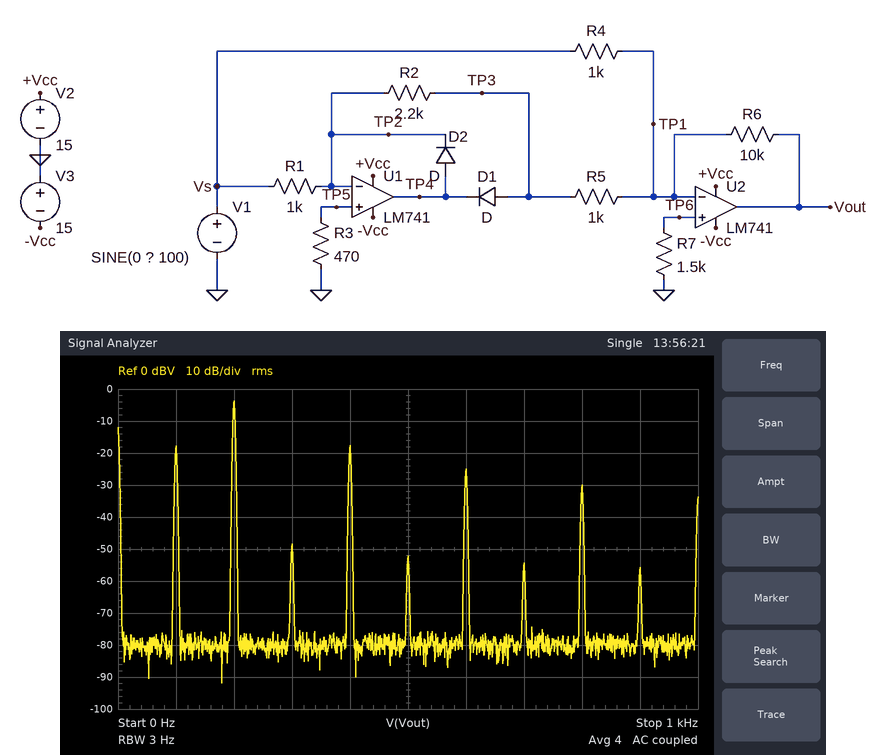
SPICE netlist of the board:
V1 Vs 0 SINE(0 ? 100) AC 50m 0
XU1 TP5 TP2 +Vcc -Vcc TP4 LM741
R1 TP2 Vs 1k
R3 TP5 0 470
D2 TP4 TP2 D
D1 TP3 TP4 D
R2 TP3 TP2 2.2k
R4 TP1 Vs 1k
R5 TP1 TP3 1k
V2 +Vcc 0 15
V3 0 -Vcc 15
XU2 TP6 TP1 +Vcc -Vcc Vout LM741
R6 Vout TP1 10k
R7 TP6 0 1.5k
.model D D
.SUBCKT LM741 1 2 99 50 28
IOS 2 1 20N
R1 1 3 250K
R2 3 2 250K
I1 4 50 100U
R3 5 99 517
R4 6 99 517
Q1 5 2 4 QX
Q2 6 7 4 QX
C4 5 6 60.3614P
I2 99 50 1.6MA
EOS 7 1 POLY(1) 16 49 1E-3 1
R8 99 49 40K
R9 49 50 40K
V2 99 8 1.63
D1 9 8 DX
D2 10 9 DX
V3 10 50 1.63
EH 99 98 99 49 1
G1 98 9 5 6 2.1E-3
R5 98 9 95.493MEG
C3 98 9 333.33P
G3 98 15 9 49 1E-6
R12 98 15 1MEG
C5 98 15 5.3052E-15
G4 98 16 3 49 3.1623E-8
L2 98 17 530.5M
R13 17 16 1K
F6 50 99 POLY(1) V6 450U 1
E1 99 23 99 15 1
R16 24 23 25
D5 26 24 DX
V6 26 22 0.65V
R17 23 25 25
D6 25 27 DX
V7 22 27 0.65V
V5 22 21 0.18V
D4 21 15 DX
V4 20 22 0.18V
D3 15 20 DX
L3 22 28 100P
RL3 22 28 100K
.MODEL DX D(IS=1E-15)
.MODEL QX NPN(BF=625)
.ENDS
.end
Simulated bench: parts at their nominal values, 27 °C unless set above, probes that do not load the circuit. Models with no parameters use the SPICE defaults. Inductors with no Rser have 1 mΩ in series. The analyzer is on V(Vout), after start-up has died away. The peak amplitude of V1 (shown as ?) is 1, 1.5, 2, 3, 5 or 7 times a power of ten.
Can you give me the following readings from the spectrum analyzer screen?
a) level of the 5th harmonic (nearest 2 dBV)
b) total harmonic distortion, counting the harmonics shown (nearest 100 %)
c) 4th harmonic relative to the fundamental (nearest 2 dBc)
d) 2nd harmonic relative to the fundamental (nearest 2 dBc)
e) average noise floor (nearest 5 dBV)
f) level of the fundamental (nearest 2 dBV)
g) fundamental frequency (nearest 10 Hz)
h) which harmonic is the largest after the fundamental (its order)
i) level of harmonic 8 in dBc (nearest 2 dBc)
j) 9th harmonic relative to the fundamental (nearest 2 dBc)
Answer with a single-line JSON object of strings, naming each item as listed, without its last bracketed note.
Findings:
{"level of the 5th harmonic": "-52 dBV", "total harmonic distortion, counting the harmonics shown": "500 %", "4th harmonic relative to the fundamental": "0 dBc", "2nd harmonic relative to the fundamental": "14 dBc", "average noise floor": "-80 dBV", "level of the fundamental": "-18 dBV", "fundamental frequency": "100 Hz", "which harmonic is the largest after the fundamental": "2", "level of harmonic 8 in dBc": "-12 dBc", "9th harmonic relative to the fundamental": "-38 dBc"}
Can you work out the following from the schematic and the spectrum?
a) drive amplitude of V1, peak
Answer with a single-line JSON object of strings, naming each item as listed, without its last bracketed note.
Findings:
{"drive amplitude of V1, peak": "200 mV"}
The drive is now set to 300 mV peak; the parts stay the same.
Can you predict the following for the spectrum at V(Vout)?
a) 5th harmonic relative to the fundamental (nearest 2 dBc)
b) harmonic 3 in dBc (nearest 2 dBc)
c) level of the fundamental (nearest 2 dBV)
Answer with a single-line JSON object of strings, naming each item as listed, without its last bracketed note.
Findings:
{"5th harmonic relative to the fundamental": "-38 dBc", "harmonic 3 in dBc": "-34 dBc", "level of the fundamental": "-14 dBV"}
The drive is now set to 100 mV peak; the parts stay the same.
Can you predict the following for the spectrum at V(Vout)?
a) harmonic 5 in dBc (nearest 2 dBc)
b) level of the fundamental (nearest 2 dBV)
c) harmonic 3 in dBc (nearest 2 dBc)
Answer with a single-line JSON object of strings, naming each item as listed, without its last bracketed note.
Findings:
{"harmonic 5 in dBc": "-28 dBc", "level of the fundamental": "-24 dBV", "harmonic 3 in dBc": "-24 dBc"}
